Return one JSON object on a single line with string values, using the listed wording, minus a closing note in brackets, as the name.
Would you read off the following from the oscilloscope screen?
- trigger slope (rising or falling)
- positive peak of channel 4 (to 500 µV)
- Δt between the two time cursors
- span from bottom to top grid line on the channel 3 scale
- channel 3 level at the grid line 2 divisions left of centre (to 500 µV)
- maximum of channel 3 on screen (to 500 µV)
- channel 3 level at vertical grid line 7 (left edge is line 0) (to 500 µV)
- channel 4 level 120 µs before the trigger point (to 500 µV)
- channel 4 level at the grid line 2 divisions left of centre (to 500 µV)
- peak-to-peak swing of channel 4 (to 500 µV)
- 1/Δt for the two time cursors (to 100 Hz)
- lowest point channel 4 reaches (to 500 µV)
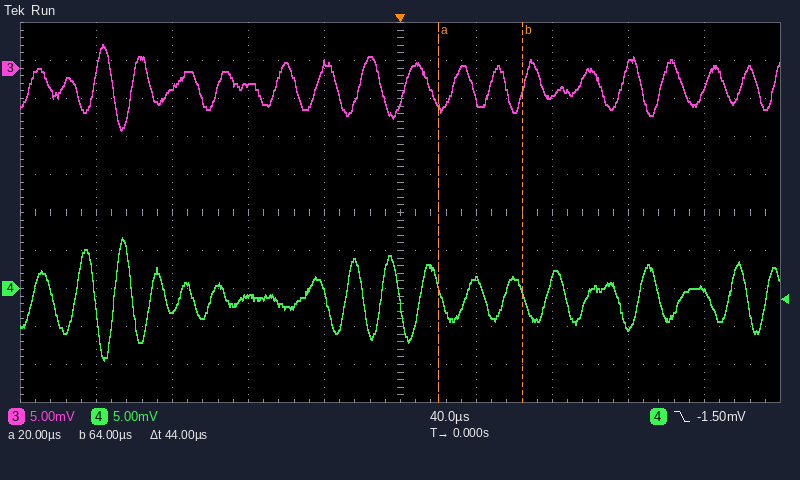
{"trigger slope": "falling", "positive peak of channel 4": "6.5 mV", "Δt between the two time cursors": "44 µs", "span from bottom to top grid line on the channel 3 scale": "50 mV", "channel 3 level at the grid line 2 divisions left of centre": "-2.0 mV", "maximum of channel 3 on screen": "3.0 mV", "channel 3 level at vertical grid line 7 (left edge is line 0)": "-3.5 mV", "channel 4 level 120 µs before the trigger point": "-3.0 mV", "channel 4 level at the grid line 2 divisions left of centre": "-1.0 mV", "peak-to-peak swing of channel 4": "16.0 mV", "1/Δt for the two time cursors": "22.7 kHz", "lowest point channel 4 reaches": "-9.5 mV"}
